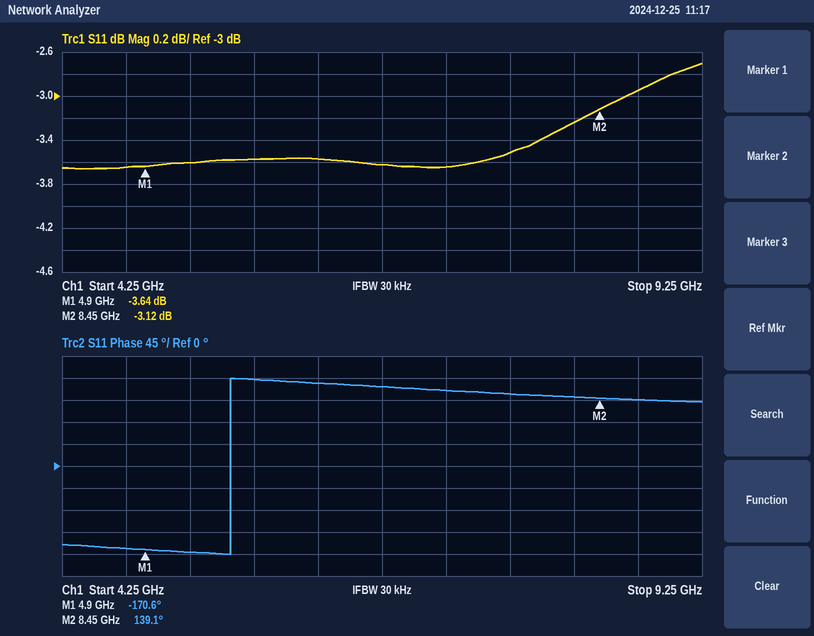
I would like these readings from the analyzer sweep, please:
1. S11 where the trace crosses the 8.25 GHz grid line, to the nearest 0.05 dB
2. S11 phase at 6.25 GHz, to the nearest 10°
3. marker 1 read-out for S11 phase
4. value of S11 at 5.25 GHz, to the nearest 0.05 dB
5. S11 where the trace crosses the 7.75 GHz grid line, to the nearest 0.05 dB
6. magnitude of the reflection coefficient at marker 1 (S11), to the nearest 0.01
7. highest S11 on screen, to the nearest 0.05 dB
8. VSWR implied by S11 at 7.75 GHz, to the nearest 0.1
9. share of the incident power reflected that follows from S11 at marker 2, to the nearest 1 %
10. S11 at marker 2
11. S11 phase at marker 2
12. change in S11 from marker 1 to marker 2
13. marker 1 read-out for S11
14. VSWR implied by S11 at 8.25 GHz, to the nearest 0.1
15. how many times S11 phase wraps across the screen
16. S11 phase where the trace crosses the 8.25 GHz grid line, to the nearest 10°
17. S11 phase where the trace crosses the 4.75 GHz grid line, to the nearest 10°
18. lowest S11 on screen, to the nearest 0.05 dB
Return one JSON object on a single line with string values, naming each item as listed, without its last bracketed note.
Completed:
{"S11 where the trace crosses the 8.25 GHz grid line, to the nearest 0.05 dB": "-3.25 dB", "S11 phase at 6.25 GHz, to the nearest 10°": "170°", "marker 1 read-out for S11 phase": "-170.6°", "value of S11 at 5.25 GHz, to the nearest 0.05 dB": "-3.60 dB", "S11 where the trace crosses the 7.75 GHz grid line, to the nearest 0.05 dB": "-3.50 dB", "magnitude of the reflection coefficient at marker 1 (S11), to the nearest 0.01": "0.66", "highest S11 on screen, to the nearest 0.05 dB": "-2.70 dB", "VSWR implied by S11 at 7.75 GHz, to the nearest 0.1": "5.0", "share of the incident power reflected that follows from S11 at marker 2, to the nearest 1 %": "49 %", "S11 at marker 2": "-3.12 dB", "S11 phase at marker 2": "139.1°", "change in S11 from marker 1 to marker 2": "0.52 dB", "marker 1 read-out for S11": "-3.64 dB", "VSWR implied by S11 at 8.25 GHz, to the nearest 0.1": "5.4", "how many times S11 phase wraps across the screen": "1", "S11 phase where the trace crosses the 8.25 GHz grid line, to the nearest 10°": "140°", "S11 phase where the trace crosses the 4.75 GHz grid line, to the nearest 10°": "-170°", "lowest S11 on screen, to the nearest 0.05 dB": "-3.65 dB"}
